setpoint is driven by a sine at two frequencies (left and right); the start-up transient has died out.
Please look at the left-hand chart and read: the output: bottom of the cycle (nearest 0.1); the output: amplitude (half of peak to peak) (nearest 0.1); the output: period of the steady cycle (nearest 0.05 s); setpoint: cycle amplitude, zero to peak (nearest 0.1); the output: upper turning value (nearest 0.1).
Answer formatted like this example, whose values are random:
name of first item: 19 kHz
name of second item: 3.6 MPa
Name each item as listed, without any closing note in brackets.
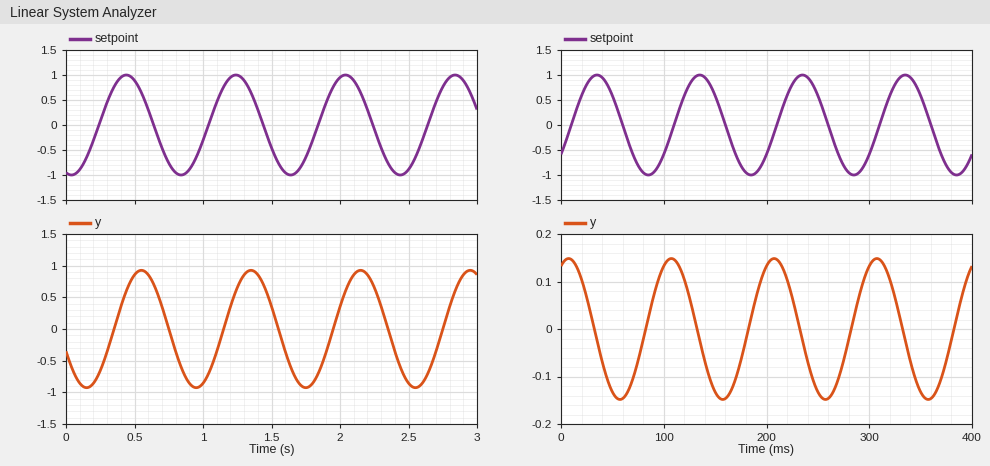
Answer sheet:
the output: bottom of the cycle: -0.9
the output: amplitude (half of peak to peak): 0.9
the output: period of the steady cycle: 0.80 s
setpoint: cycle amplitude, zero to peak: 1.0
the output: upper turning value: 0.9
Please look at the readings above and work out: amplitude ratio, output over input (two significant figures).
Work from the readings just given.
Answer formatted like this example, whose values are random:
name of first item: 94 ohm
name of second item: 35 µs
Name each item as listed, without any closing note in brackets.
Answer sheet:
amplitude ratio, output over input: 0.90
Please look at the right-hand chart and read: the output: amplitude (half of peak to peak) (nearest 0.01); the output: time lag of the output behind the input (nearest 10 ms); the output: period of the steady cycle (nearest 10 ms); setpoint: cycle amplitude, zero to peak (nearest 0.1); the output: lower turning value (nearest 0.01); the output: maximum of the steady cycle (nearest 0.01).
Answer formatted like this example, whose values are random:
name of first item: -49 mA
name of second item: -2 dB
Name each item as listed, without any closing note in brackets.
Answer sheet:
the output: amplitude (half of peak to peak): 0.15
the output: time lag of the output behind the input: 70 ms
the output: period of the steady cycle: 100 ms
setpoint: cycle amplitude, zero to peak: 1.0
the output: lower turning value: -0.15
the output: maximum of the steady cycle: 0.15
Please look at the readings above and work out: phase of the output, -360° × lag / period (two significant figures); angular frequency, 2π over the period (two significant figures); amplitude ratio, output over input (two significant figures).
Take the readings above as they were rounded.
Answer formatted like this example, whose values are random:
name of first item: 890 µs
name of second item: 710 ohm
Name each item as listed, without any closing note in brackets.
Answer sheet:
phase of the output, -360° × lag / period: -250°
angular frequency, 2π over the period: 0.063 rad/ms
amplitude ratio, output over input: 0.15
